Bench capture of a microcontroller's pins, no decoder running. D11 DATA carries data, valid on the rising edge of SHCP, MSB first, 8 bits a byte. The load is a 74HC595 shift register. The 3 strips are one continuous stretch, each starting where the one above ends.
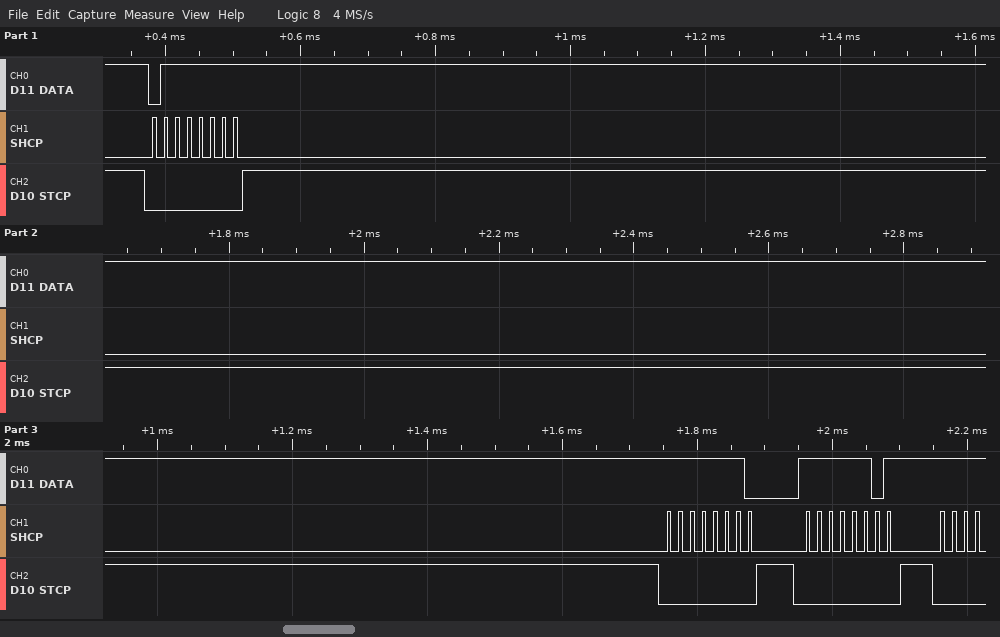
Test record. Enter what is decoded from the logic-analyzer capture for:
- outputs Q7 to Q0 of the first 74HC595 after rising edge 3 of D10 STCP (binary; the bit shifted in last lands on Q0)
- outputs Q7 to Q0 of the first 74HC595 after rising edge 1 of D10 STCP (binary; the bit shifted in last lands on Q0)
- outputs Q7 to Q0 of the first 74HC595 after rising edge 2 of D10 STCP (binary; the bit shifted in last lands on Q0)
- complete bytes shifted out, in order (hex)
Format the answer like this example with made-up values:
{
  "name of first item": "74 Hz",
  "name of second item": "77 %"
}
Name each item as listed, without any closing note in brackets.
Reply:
{
  "outputs Q7 to Q0 of the first 74HC595 after rising edge 3 of D10 STCP": "11111101",
  "outputs Q7 to Q0 of the first 74HC595 after rising edge 1 of D10 STCP": "01111111",
  "outputs Q7 to Q0 of the first 74HC595 after rising edge 2 of D10 STCP": "11111110",
  "complete bytes shifted out, in order": "7F FE FD"
}
